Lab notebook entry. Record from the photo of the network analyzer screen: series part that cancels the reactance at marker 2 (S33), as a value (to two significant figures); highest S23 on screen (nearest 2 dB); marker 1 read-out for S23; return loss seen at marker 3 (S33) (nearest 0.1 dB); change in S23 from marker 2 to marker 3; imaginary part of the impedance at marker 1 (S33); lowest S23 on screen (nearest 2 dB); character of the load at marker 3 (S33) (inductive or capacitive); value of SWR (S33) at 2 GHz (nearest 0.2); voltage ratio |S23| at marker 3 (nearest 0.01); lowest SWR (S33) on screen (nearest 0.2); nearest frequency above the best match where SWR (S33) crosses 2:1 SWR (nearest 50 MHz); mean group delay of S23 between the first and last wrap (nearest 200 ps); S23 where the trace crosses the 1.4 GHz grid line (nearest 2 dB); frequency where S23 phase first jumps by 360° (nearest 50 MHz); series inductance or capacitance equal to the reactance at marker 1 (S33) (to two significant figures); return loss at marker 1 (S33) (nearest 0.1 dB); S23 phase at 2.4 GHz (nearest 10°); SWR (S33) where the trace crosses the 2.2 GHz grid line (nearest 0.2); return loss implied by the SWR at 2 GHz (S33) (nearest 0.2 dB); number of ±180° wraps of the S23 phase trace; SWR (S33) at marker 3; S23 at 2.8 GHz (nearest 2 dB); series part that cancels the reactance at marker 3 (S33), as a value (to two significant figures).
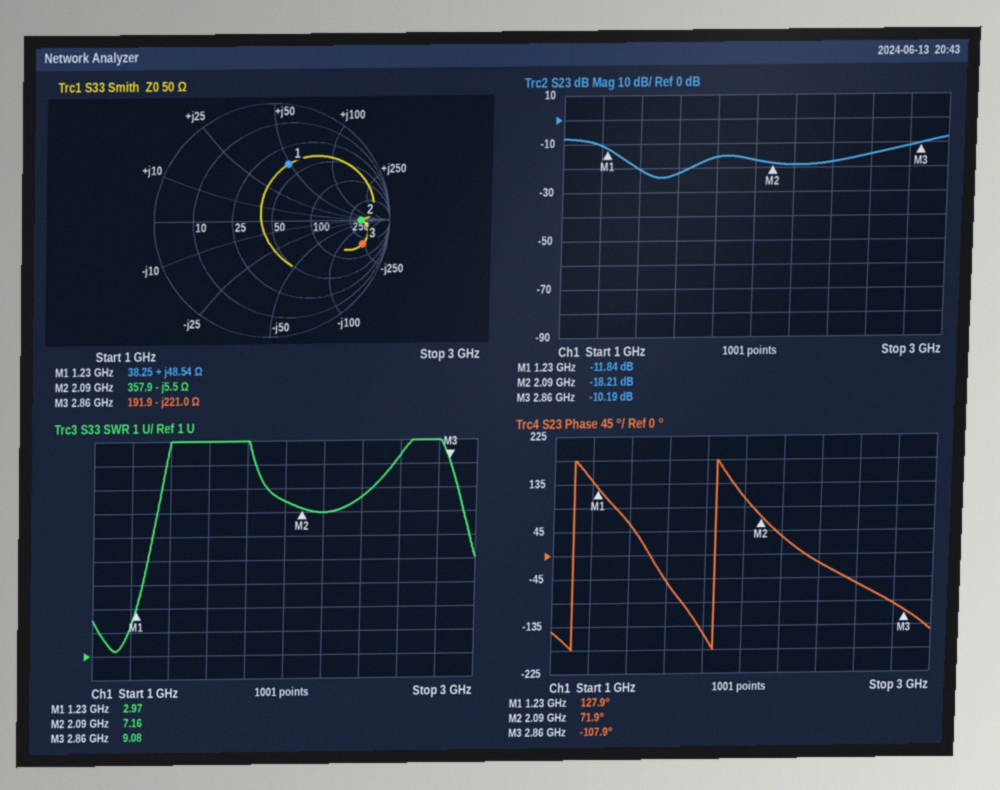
420 pH
-8 dB
-11.84 dB
1.9 dB
8.02 dB
+48.54 Ω
-24 dB
capacitive
7.4
0.31
1.2
1.20 GHz
1.4 ns
-20 dB
1.10 GHz
6.3 nH
6.1 dB
-20°
7.0
2.4 dB
2
9.08
-12 dB
12 nH
